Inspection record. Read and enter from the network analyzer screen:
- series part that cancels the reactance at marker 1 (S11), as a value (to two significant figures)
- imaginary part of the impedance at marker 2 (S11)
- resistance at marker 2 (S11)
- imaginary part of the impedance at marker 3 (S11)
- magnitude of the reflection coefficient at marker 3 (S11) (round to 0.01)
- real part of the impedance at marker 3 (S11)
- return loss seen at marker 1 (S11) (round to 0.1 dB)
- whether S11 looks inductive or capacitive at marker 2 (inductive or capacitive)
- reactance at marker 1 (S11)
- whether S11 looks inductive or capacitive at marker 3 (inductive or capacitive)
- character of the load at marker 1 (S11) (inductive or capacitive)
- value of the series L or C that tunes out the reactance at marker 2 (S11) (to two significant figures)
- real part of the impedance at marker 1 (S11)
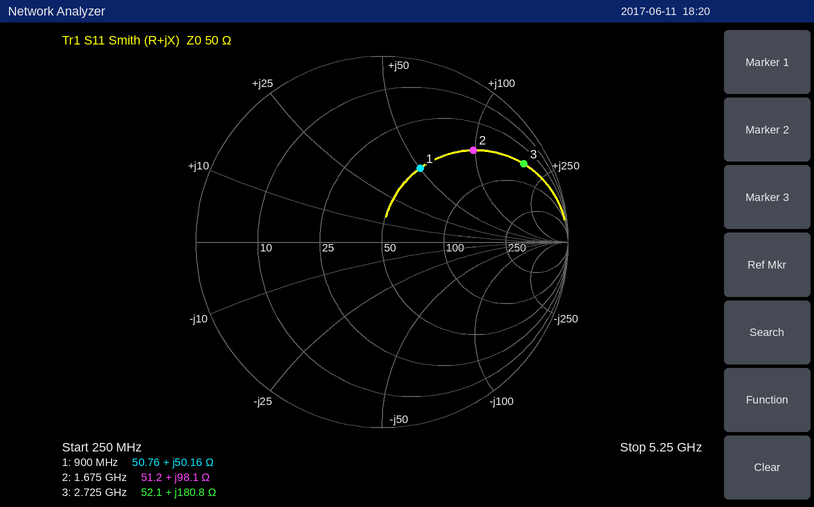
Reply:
3.5 pF
+98.1 Ω
51.2 Ω
+180.8 Ω
0.87
52.1 Ω
7.0 dB
inductive
+50.16 Ω
inductive
inductive
970 fF
50.76 Ω
